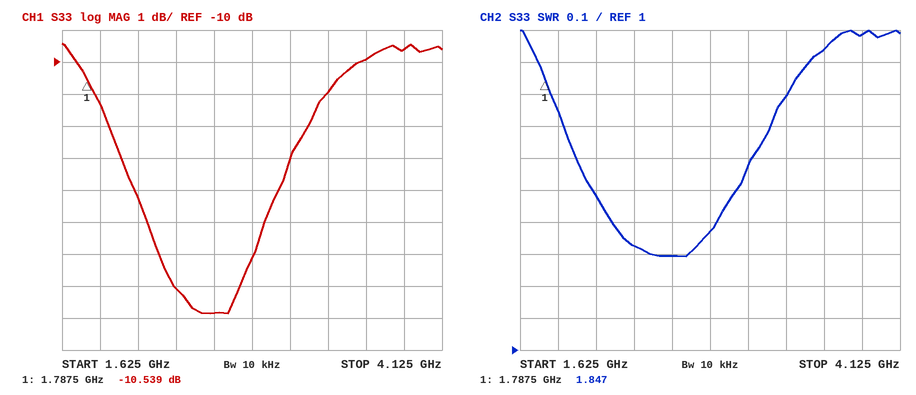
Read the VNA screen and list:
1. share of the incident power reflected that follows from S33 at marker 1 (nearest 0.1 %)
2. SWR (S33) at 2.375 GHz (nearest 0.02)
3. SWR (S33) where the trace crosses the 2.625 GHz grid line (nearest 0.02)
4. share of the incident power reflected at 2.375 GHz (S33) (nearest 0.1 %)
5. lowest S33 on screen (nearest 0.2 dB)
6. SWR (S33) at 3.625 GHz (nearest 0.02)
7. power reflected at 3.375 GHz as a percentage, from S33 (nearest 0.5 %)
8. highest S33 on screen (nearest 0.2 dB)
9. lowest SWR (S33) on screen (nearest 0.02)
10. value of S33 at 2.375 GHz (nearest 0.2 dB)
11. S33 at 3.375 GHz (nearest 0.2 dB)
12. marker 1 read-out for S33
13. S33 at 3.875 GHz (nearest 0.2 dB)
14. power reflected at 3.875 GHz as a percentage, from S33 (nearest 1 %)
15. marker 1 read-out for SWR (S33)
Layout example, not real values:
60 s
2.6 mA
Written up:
8.8 %
1.32
1.30
2.0 %
-17.8 dB
1.94
8.0 %
-9.4 dB
1.30
-17.0 dB
-11.0 dB
-10.539 dB
-9.6 dB
11 %
1.847
